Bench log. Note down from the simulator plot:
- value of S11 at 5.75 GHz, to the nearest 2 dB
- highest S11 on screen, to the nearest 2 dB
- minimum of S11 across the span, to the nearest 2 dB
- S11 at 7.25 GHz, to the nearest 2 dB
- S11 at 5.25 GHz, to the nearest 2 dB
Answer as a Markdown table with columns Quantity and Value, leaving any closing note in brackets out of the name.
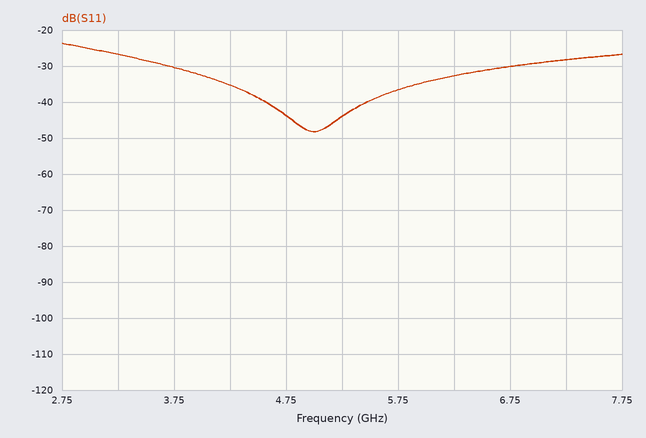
| Quantity | Value |
|---|---|
| value of S11 at 5.75 GHz, to the nearest 2 dB | -36 dB |
| highest S11 on screen, to the nearest 2 dB | -24 dB |
| minimum of S11 across the span, to the nearest 2 dB | -48 dB |
| S11 at 7.25 GHz, to the nearest 2 dB | -28 dB |
| S11 at 5.25 GHz, to the nearest 2 dB | -44 dB |
